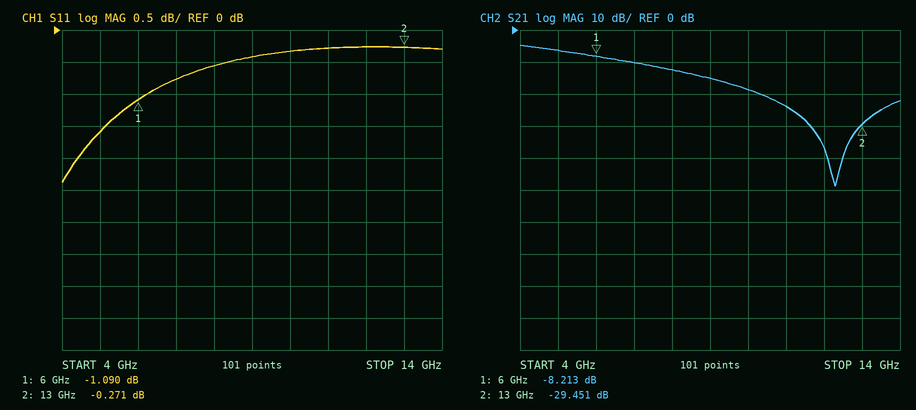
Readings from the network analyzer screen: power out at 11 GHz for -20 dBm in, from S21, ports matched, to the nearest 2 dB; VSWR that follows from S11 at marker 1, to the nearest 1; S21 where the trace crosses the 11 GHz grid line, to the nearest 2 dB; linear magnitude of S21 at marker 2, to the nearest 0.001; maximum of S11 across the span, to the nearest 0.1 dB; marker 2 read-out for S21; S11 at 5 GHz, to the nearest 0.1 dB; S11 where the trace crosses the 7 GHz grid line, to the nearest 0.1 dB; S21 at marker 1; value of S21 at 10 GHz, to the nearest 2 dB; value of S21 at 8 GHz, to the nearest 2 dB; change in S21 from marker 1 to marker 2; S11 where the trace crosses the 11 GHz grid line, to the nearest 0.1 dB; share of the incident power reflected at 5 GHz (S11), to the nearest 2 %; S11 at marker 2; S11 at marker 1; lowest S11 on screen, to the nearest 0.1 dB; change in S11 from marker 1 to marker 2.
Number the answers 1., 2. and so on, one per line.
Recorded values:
1. -44 dBm
2. 16
3. -24 dB
4. 0.034
5. -0.3 dB
6. -29.451 dB
7. -1.6 dB
8. -0.8 dB
9. -8.213 dB
10. -18 dB
11. -12 dB
12. -21.238 dB
13. -0.3 dB
14. 70 %
15. -0.271 dB
16. -1.090 dB
17. -2.4 dB
18. 0.819 dB
